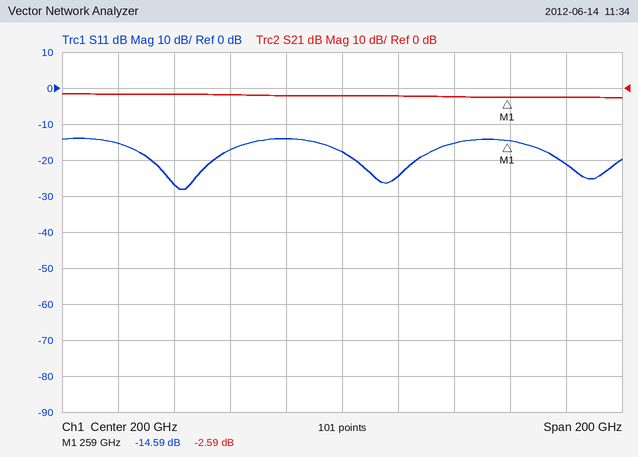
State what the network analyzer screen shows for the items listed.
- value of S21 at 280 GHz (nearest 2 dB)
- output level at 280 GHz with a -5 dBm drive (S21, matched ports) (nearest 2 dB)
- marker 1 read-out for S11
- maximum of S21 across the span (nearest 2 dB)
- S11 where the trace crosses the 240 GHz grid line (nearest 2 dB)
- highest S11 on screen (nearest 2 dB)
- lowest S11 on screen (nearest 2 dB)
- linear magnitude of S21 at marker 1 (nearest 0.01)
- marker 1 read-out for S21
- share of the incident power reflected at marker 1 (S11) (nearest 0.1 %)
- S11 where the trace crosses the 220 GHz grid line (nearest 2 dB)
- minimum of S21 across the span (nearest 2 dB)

-2 dB
-8 dBm
-14.59 dB
-2 dB
-16 dB
-14 dB
-28 dB
0.74
-2.59 dB
3.5 %
-24 dB
-2 dB
